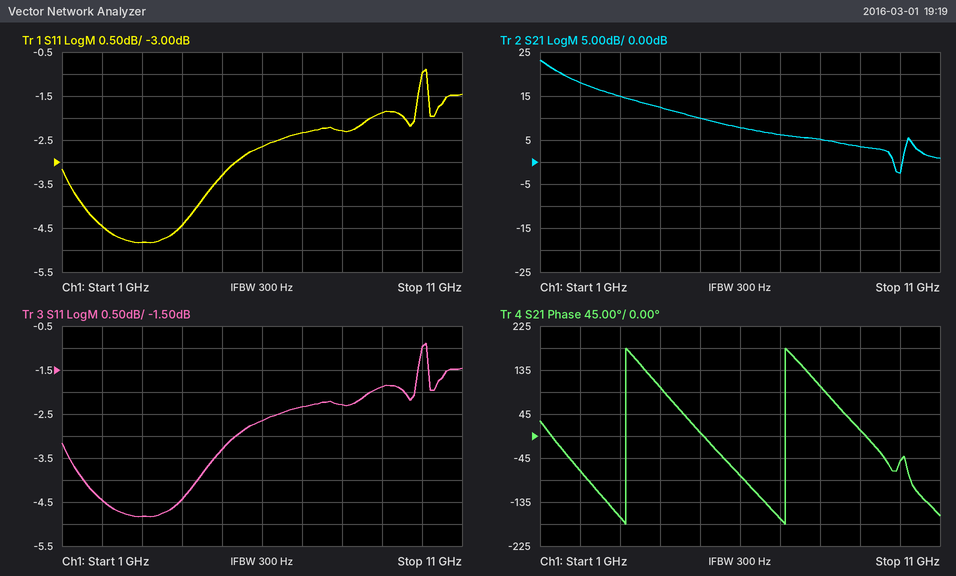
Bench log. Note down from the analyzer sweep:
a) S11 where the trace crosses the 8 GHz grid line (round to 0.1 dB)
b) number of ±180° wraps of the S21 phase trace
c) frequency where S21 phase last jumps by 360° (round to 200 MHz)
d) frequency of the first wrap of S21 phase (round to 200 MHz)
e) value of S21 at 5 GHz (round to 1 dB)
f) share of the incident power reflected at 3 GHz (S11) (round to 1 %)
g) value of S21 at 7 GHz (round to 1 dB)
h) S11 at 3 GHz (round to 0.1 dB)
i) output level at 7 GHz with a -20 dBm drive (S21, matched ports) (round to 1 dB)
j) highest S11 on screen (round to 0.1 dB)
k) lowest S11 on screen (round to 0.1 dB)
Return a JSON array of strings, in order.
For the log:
["-2.3 dB", "2", "7.2 GHz", "3.2 GHz", "10 dB", "33 %", "6 dB", "-4.8 dB", "-14 dBm", "-0.9 dB", "-4.8 dB"]
